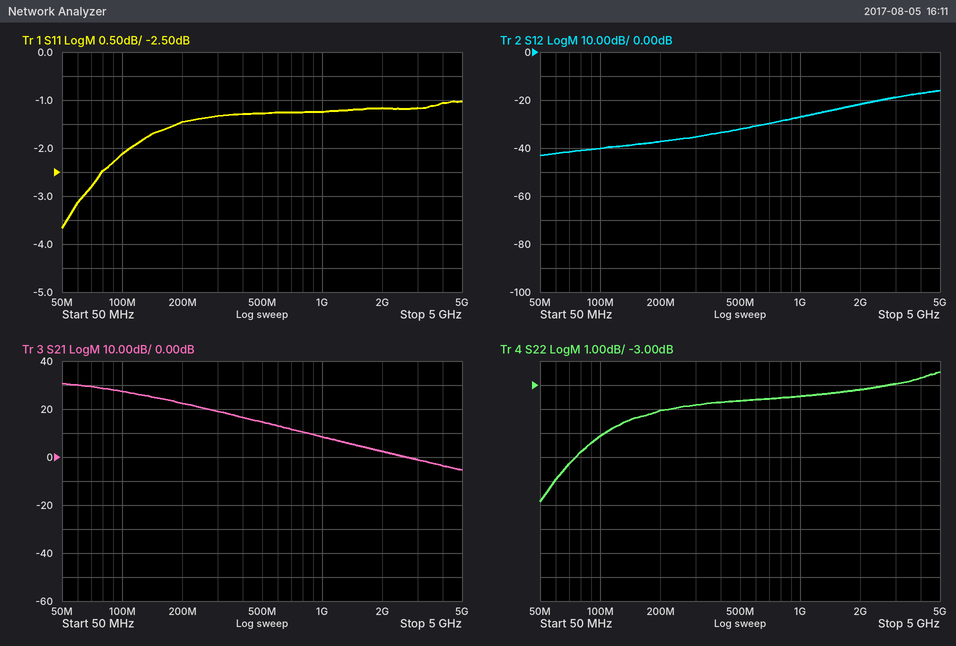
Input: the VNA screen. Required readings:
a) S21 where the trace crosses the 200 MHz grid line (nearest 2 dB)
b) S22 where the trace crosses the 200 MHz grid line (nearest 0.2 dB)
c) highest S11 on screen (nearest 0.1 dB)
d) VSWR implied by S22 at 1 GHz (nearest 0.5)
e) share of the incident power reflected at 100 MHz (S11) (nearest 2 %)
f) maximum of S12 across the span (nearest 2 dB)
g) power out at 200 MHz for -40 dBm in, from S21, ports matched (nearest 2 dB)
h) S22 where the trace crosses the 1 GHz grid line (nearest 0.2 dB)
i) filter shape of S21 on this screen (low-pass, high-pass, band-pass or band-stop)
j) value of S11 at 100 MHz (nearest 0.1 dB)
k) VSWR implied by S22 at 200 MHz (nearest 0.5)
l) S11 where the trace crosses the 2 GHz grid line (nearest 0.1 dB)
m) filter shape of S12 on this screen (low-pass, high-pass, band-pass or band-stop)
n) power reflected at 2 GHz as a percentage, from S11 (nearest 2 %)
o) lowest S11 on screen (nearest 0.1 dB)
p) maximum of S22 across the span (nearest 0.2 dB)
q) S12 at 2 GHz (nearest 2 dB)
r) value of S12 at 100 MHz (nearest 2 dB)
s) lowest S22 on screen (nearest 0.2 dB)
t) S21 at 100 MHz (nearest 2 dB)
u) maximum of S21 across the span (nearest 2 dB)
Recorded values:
22 dB
-4.0 dB
-1.0 dB
5.0
62 %
-16 dB
-18 dBm
-3.4 dB
low-pass
-2.1 dB
4.5
-1.2 dB
high-pass
76 %
-3.7 dB
-2.4 dB
-22 dB
-40 dB
-7.8 dB
28 dB
30 dB
